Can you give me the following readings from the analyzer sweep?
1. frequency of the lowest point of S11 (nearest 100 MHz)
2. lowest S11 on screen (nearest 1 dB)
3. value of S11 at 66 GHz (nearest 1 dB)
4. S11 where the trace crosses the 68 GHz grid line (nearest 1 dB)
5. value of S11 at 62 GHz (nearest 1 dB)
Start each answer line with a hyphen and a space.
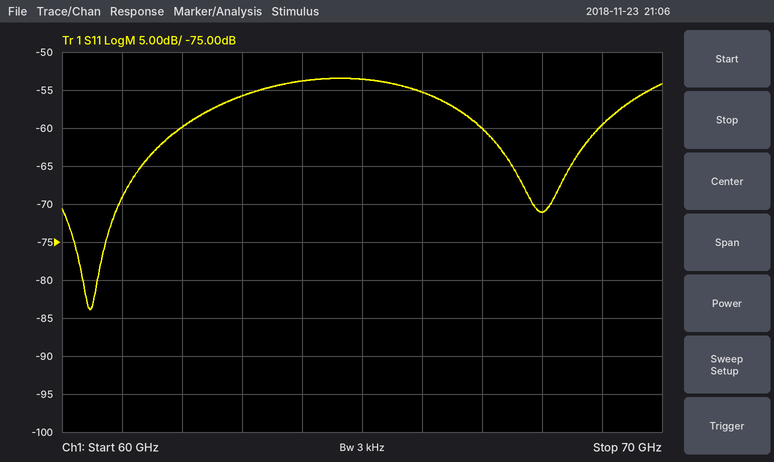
- 60.5 GHz
- -84 dB
- -55 dB
- -71 dB
- -60 dB
